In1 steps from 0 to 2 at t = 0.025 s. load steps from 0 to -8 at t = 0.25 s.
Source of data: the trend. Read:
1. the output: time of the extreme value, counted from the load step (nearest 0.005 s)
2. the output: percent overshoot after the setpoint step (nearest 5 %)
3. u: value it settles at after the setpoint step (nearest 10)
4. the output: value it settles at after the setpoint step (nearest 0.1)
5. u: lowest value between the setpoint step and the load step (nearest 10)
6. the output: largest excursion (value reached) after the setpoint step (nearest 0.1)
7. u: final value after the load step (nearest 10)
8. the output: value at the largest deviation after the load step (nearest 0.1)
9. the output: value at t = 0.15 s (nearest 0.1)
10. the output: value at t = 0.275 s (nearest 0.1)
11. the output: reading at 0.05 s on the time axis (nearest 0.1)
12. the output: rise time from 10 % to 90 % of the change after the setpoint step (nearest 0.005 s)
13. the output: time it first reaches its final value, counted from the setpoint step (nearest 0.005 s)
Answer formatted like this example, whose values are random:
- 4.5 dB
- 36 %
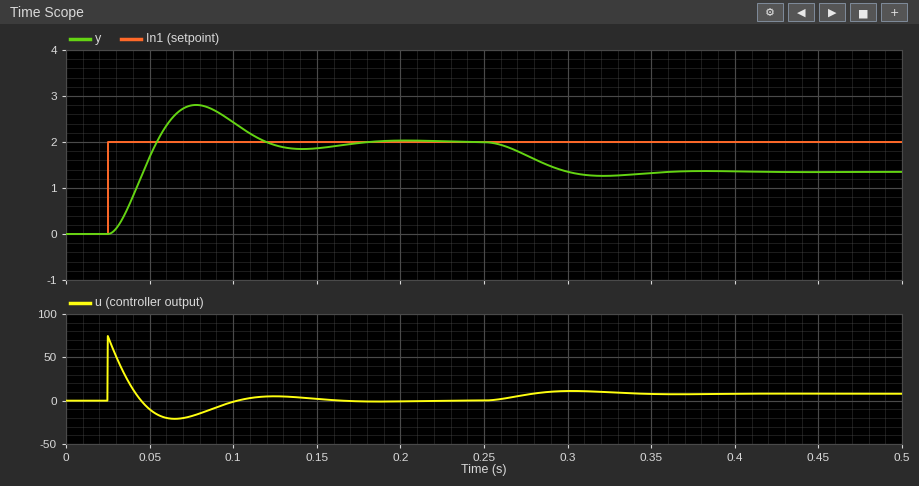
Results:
- 0.070 s
- 40 %
- 0
- 2.0
- -20
- 2.8
- 10
- 1.3
- 1.9
- 1.7
- 1.7
- 0.020 s
- 0.030 s
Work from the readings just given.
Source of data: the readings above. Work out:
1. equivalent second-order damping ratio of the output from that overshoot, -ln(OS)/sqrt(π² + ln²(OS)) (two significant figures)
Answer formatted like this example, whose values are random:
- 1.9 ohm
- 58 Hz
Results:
- 0.28
